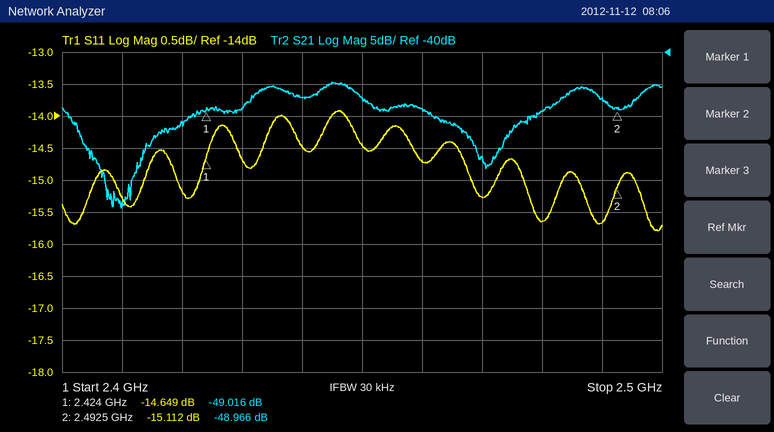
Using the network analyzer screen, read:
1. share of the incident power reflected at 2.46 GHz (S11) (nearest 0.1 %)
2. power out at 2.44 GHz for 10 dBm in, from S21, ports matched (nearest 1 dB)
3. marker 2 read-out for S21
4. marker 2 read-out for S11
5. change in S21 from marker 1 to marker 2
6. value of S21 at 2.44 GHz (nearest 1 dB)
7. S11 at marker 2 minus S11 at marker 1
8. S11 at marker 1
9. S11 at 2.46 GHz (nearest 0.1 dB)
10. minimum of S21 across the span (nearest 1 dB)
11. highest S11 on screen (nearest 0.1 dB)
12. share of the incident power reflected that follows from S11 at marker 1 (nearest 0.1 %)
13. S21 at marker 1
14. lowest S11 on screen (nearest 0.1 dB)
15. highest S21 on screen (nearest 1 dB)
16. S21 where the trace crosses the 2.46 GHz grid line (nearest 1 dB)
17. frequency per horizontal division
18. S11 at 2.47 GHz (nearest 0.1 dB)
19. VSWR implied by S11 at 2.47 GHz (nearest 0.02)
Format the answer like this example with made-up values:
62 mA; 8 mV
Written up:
3.4 %; -37 dBm; -48.966 dB; -15.112 dB; 0.050 dB; -47 dB; -0.463 dB; -14.649 dB; -14.7 dB; -64 dB; -13.9 dB; 3.4 %; -49.016 dB; -15.8 dB; -45 dB; -49 dB; 10 MHz; -15.3 dB; 1.42
